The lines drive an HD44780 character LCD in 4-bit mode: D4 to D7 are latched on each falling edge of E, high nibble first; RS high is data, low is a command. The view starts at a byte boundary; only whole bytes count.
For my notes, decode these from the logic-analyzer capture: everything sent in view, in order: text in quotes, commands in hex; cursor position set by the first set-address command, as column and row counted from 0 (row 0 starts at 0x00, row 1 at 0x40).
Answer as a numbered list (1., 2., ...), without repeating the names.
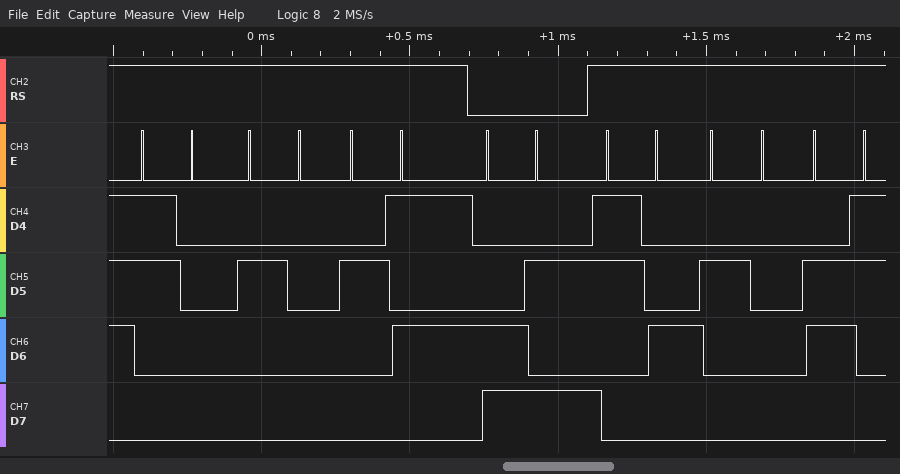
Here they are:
1. "0 %" 0xCA "4 c"
2. column 10, row 1
